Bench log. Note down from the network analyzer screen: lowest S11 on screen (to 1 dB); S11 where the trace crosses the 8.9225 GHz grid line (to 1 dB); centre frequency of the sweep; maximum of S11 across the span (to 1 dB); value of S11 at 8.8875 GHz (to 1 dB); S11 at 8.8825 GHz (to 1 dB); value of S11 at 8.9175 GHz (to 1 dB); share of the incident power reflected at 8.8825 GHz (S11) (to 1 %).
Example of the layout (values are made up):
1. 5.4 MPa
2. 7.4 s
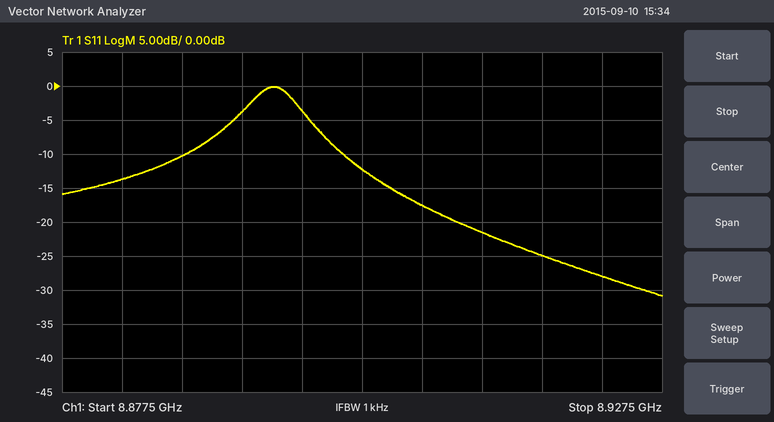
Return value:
1. -31 dB
2. -28 dB
3. 8.9025 GHz
4. 0 dB
5. -10 dB
6. -14 dB
7. -25 dB
8. 4 %
